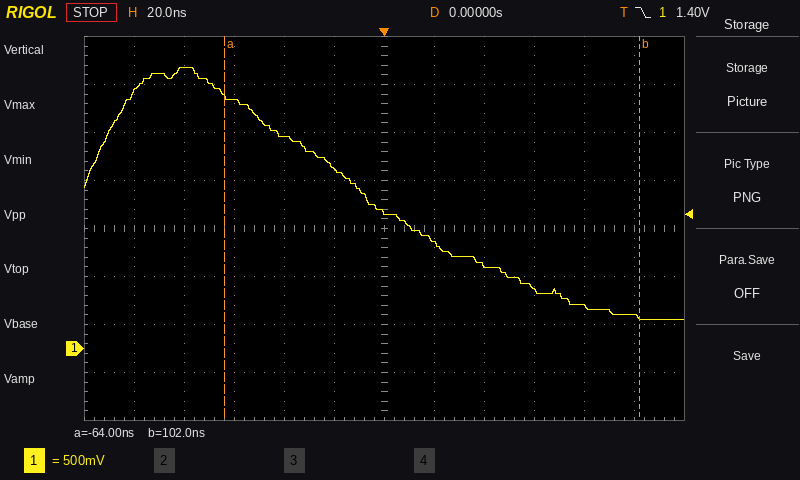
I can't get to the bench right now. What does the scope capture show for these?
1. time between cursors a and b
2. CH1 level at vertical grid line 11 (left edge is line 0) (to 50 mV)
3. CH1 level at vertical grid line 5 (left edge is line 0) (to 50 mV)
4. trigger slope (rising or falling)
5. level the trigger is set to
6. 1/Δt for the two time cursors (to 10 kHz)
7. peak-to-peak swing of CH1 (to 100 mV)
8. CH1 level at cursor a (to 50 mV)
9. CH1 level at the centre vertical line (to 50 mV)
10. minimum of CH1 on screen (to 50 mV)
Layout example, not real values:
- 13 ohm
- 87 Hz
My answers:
- 166 ns
- 350 mV
- 1.85 V
- falling
- 1.40 V
- 6.02 MHz
- 2.60 V
- 2.65 V
- 1.40 V
- 300 mV
